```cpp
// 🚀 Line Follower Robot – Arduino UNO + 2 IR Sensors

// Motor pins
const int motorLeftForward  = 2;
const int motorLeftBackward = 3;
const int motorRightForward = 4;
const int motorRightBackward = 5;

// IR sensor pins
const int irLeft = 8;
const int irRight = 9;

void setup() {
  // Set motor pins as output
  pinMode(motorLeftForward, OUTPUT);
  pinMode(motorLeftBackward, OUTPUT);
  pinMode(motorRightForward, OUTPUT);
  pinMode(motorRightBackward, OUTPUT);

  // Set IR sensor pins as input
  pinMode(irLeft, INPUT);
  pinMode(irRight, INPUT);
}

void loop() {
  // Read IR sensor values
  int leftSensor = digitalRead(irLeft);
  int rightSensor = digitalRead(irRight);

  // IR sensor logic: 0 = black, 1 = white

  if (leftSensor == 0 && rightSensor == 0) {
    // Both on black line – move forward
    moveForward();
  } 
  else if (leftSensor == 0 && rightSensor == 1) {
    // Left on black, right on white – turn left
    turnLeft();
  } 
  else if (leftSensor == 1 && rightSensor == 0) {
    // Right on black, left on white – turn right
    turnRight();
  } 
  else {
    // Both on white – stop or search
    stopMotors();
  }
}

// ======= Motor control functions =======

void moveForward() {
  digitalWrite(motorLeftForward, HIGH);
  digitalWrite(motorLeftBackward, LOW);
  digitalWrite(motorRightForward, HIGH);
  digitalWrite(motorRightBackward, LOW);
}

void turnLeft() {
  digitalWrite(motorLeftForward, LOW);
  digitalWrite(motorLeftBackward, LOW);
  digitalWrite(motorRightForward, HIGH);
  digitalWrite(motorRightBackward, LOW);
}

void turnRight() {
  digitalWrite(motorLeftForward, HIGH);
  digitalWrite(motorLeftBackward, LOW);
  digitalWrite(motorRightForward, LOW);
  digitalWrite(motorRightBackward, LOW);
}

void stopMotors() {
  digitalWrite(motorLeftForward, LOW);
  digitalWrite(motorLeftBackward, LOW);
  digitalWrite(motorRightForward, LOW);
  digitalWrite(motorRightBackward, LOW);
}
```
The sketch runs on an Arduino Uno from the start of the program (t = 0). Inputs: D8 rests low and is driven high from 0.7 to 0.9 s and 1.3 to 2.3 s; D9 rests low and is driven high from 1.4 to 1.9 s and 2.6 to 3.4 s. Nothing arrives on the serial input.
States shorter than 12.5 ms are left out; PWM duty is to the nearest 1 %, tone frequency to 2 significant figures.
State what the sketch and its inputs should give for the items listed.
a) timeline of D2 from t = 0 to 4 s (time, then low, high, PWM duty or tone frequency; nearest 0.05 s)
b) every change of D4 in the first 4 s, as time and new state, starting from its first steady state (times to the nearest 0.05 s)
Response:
0 s high; 1.4 s low; 1.9 s high; 2.6 s low; 3.4 s high
0 s high; 0.7 s low; 0.9 s high; 1.3 s low; 2.3 s high
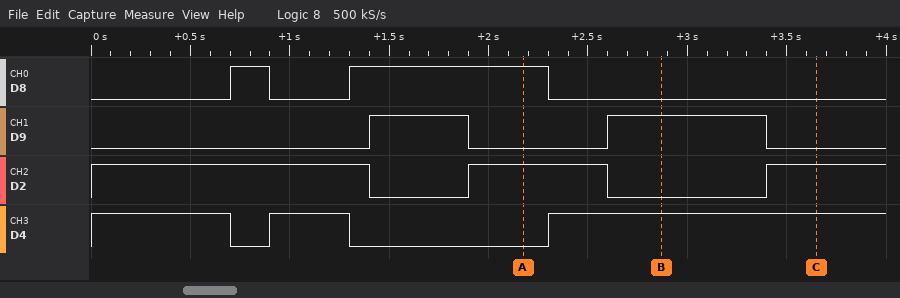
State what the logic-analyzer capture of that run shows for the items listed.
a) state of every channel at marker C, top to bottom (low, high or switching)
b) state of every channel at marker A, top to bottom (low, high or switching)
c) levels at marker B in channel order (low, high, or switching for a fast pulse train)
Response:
D8 low, D9 low, D2 high, D4 high
D8 high, D9 low, D2 high, D4 low
D8 low, D9 high, D2 low, D4 high
